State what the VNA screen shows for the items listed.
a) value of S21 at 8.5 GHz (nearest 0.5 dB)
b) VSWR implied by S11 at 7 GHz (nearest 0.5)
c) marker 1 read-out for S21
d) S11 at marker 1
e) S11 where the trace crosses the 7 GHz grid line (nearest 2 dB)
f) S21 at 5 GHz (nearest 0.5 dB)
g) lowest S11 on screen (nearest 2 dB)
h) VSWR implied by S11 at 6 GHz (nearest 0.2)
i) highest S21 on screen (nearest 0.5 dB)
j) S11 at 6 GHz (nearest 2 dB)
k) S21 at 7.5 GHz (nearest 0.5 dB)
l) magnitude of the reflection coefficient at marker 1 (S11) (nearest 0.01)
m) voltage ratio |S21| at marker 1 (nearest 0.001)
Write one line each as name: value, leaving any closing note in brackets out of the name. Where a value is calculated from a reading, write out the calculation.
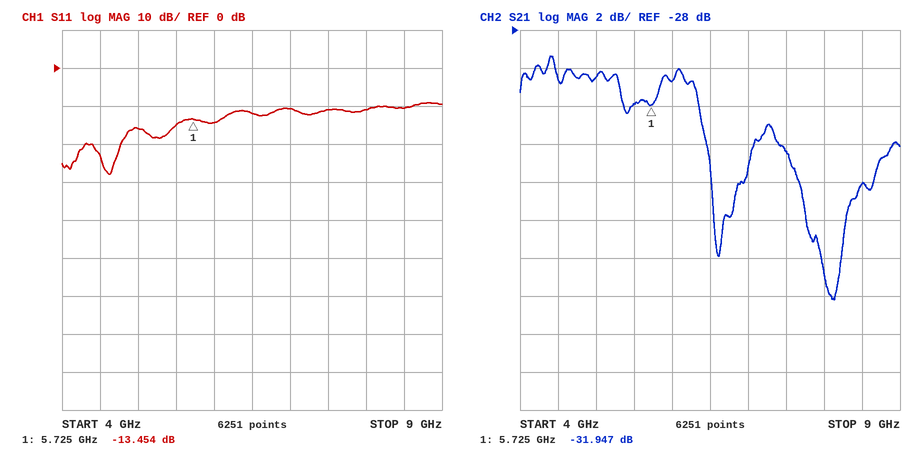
value of S21 at 8.5 GHz: -36.0 dB
VSWR implied by S11 at 7 GHz: |Γ| = 10^(-10/20) = 0.3162; VSWR = (1 + 0.3162)/(1 − 0.3162) ≈ 1.92, so 2.0 to the nearest 0.5
marker 1 read-out for S21: -31.947 dB
S11 at marker 1: -13.454 dB
S11 where the trace crosses the 7 GHz grid line: -10 dB
S21 at 5 GHz: -30.5 dB
lowest S11 on screen: -28 dB
VSWR implied by S11 at 6 GHz: |Γ| = 10^(-14/20) = 0.1995; VSWR = (1 + 0.1995)/(1 − 0.1995) ≈ 1.50, so 1.4 to the nearest 0.2
highest S21 on screen: -29.5 dB
S11 at 6 GHz: -14 dB
S21 at 7.5 GHz: -34.5 dB
magnitude of the reflection coefficient at marker 1 (S11): 10^(-13.454/20) ≈ 0.21
voltage ratio |S21| at marker 1: 10^(-31.947/20) ≈ 0.025
